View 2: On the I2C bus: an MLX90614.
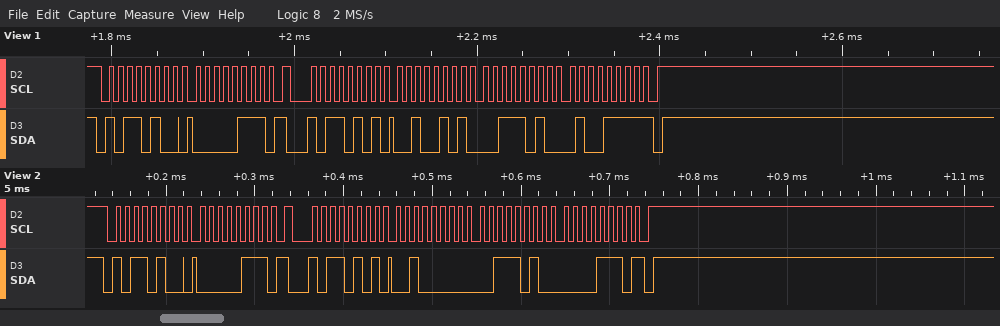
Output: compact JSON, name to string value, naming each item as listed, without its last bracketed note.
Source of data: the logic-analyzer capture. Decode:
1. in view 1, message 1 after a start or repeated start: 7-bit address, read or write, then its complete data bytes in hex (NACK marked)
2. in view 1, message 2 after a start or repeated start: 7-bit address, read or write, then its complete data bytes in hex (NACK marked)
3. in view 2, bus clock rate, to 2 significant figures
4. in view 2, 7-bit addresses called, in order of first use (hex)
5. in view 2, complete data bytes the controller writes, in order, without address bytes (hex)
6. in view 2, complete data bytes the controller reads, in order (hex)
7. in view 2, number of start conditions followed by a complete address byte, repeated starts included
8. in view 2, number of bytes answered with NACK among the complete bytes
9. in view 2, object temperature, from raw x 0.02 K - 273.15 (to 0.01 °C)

{"in view 1, message 1 after a start or repeated start: 7-bit address, read or write, then its complete data bytes in hex": "0x5A write: 07", "in view 1, message 2 after a start or repeated start: 7-bit address, read or write, then its complete data bytes in hex": "0x5A read: 25 3A 4F NACK", "in view 2, bus clock rate, to 2 significant figures": "100 kHz", "in view 2, 7-bit addresses called, in order of first use": "0x5A", "in view 2, complete data bytes the controller writes, in order, without address bytes": "07", "in view 2, complete data bytes the controller reads, in order": "20 3A 0E", "in view 2, number of start conditions followed by a complete address byte, repeated starts included": "2", "in view 2, number of bytes answered with NACK among the complete bytes": "1", "in view 2, object temperature, from raw x 0.02 K - 273.15": "24.45 °C"}
